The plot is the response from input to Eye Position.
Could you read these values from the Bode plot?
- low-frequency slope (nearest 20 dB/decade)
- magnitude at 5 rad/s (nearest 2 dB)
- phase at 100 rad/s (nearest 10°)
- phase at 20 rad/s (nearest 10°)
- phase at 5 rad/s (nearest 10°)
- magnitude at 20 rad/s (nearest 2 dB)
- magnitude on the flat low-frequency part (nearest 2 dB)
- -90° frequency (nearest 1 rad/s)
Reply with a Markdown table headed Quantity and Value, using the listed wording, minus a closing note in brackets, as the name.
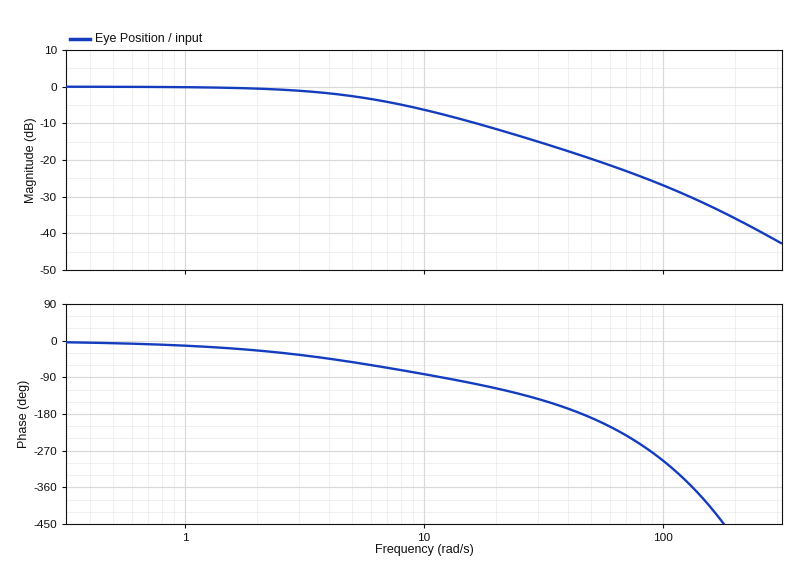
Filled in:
| Quantity | Value |
|---|---|
| low-frequency slope | 0 dB/decade |
| magnitude at 5 rad/s | -2 dB |
| phase at 100 rad/s | -290° |
| phase at 20 rad/s | -120° |
| phase at 5 rad/s | -50° |
| magnitude at 20 rad/s | -12 dB |
| magnitude on the flat low-frequency part | 0 dB |
| -90° frequency | 12 rad/s |
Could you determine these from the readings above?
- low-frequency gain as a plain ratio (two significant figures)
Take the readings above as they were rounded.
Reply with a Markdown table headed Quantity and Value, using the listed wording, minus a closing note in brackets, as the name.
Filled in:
| Quantity | Value |
|---|---|
| low-frequency gain as a plain ratio | 1.0 |
